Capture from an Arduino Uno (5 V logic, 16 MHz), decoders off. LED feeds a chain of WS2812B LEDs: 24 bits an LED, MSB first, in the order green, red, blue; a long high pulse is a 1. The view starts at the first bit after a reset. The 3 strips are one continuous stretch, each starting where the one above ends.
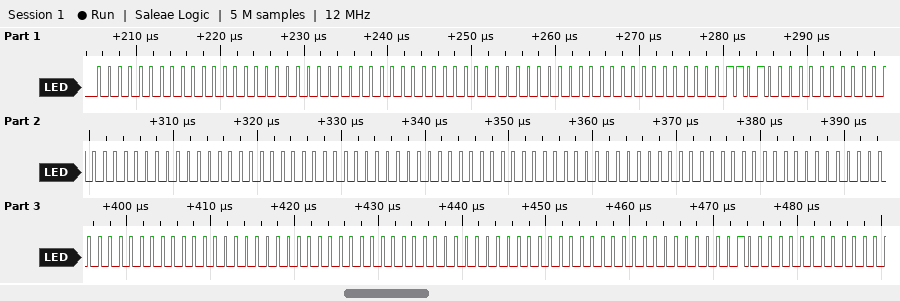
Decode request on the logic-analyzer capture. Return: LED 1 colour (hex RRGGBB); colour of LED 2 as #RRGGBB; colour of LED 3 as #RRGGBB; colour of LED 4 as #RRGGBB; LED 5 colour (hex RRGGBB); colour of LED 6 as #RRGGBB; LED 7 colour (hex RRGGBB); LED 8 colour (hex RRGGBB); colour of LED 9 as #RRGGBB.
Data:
#000000
#000000
#0D0000
#000000
#000000
#000000
#000000
#000000
#000002
